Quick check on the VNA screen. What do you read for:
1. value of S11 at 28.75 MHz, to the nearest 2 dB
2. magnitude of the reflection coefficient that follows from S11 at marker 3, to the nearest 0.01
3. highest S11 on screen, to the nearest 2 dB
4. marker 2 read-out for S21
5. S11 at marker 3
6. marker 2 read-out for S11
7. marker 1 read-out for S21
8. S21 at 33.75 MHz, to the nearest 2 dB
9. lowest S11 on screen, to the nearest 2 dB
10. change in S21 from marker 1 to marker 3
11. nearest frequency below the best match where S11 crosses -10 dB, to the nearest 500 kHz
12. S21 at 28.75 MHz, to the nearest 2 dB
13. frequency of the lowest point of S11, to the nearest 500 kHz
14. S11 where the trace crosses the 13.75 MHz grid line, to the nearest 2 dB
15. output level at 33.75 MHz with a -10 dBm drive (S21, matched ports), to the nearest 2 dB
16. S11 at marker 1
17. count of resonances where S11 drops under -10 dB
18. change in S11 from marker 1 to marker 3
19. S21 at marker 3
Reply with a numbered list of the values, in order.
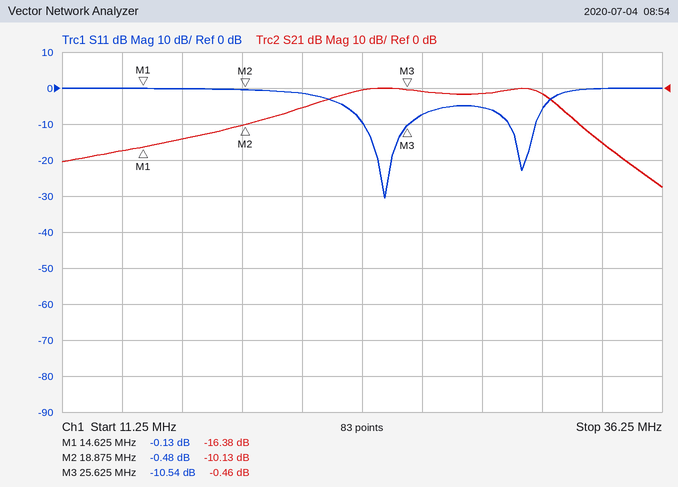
1. -6 dB
2. 0.30
3. 0 dB
4. -10.13 dB
5. -10.54 dB
6. -0.48 dB
7. -16.38 dB
8. -16 dB
9. -30 dB
10. 15.92 dB
11. 24.0 MHz
12. -2 dB
13. 24.5 MHz
14. 0 dB
15. -26 dBm
16. -0.13 dB
17. 2
18. -10.41 dB
19. -0.46 dB
